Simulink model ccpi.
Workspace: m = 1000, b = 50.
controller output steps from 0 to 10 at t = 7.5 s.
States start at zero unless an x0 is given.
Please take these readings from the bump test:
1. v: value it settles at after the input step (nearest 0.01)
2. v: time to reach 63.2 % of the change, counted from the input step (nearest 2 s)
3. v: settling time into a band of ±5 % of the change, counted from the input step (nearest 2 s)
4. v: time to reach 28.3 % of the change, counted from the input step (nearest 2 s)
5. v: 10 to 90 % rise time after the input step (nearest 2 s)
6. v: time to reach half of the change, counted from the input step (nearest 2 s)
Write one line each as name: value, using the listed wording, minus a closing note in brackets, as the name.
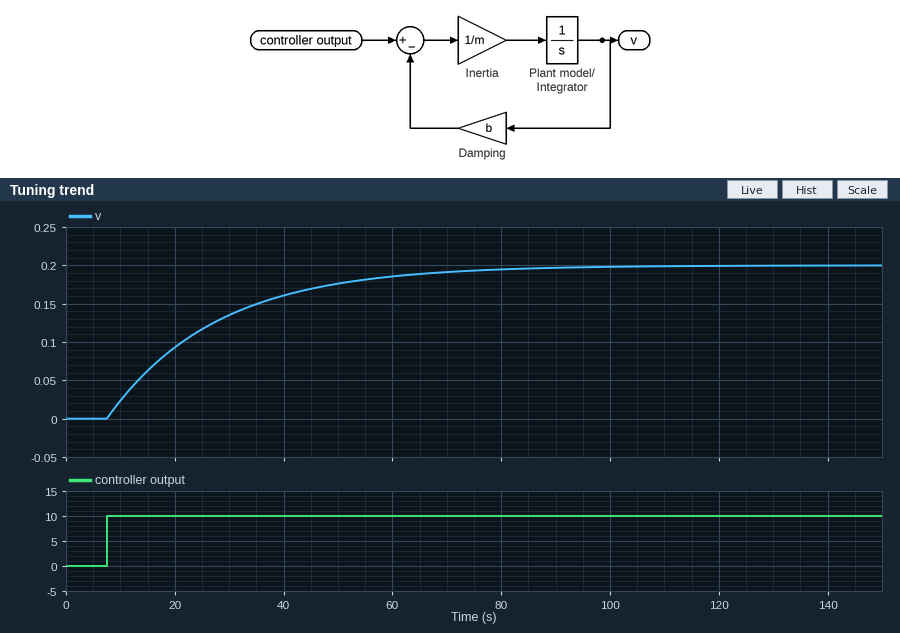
v: value it settles at after the input step: 0.20
v: time to reach 63.2 % of the change, counted from the input step: 20 s
v: settling time into a band of ±5 % of the change, counted from the input step: 60 s
v: time to reach 28.3 % of the change, counted from the input step: 6 s
v: 10 to 90 % rise time after the input step: 44 s
v: time to reach half of the change, counted from the input step: 14 s
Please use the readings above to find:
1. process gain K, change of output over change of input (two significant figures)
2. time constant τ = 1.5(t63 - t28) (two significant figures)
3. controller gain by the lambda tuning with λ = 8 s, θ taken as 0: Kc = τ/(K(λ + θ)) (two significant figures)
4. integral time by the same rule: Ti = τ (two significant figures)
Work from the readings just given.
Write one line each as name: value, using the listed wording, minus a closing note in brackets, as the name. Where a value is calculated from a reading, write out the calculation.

process gain K, change of output over change of input: (0.2 - 0) / 10 = 0.020
time constant τ = 1.5(t63 - t28): 1.5 × (20 - 6) = 21 s
controller gain by the lambda tuning with λ = 8 s, θ taken as 0: Kc = τ/(K(λ + θ)): 21 / (0.02 × (8 + 0)) = 130
integral time by the same rule: Ti = τ: 21 s
